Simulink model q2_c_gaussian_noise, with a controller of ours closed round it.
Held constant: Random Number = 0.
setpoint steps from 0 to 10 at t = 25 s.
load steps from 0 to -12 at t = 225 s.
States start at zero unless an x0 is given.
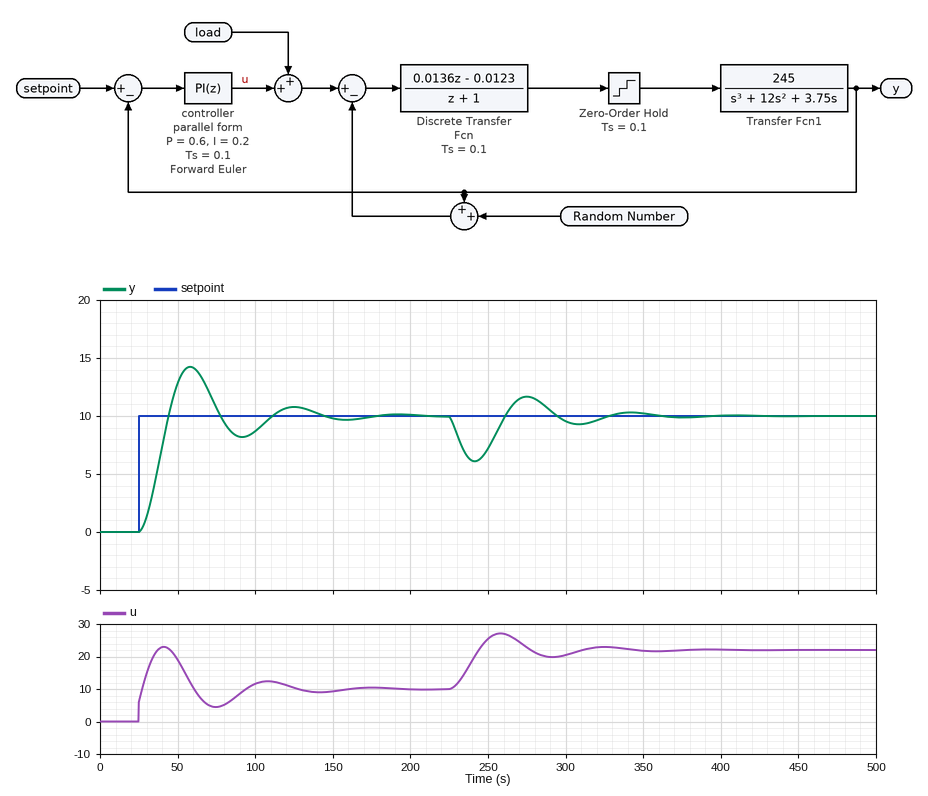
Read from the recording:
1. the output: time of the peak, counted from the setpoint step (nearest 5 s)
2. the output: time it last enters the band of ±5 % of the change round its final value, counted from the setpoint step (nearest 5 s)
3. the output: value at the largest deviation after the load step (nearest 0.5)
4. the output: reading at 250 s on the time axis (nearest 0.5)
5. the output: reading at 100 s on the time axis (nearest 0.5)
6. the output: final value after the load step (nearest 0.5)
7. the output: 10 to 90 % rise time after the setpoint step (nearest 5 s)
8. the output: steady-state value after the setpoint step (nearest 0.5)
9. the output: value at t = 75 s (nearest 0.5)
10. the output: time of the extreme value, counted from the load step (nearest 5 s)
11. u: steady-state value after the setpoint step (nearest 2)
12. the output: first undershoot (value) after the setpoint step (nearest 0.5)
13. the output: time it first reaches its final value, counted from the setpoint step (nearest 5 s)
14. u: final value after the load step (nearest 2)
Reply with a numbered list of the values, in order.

1. 35 s
2. 110 s
3. 6.0
4. 7.0
5. 8.5
6. 10.0
7. 15 s
8. 10.0
9. 10.5
10. 15 s
11. 10
12. 8.0
13. 20 s
14. 22
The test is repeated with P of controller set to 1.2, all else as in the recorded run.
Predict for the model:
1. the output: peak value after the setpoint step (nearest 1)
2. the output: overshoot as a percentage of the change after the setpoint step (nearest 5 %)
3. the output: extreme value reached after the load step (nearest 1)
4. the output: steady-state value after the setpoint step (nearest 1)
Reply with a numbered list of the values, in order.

1. 13
2. 30 %
3. 7
4. 10
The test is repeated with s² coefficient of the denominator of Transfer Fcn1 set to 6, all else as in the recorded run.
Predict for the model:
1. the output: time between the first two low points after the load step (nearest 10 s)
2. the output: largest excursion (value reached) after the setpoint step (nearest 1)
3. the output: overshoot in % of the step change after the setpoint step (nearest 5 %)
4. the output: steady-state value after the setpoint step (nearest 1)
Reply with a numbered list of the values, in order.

1. 70 s
2. 13
3. 35 %
4. 10
